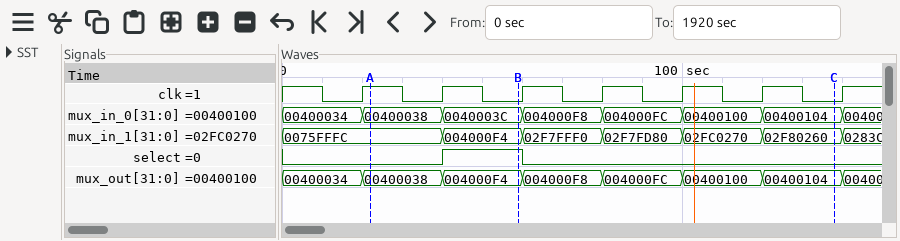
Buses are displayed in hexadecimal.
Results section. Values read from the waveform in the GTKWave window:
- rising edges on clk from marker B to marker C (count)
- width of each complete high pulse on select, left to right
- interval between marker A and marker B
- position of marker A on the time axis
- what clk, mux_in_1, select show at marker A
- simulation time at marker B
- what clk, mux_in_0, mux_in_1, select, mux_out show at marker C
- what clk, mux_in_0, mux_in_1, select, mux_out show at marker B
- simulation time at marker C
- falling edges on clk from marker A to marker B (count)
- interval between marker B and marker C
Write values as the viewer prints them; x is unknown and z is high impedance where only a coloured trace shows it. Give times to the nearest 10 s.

4
20 s
40 s
20 s
clk=1, mux_in_1=0075FFFC, select=0
60 s
clk=0, mux_in_0=00400104, mux_in_1=02F80260, select=0, mux_out=00400104
clk=0, mux_in_0=0040003C, mux_in_1=004000F4, select=1, mux_out=004000F4
140 s
2
80 s
